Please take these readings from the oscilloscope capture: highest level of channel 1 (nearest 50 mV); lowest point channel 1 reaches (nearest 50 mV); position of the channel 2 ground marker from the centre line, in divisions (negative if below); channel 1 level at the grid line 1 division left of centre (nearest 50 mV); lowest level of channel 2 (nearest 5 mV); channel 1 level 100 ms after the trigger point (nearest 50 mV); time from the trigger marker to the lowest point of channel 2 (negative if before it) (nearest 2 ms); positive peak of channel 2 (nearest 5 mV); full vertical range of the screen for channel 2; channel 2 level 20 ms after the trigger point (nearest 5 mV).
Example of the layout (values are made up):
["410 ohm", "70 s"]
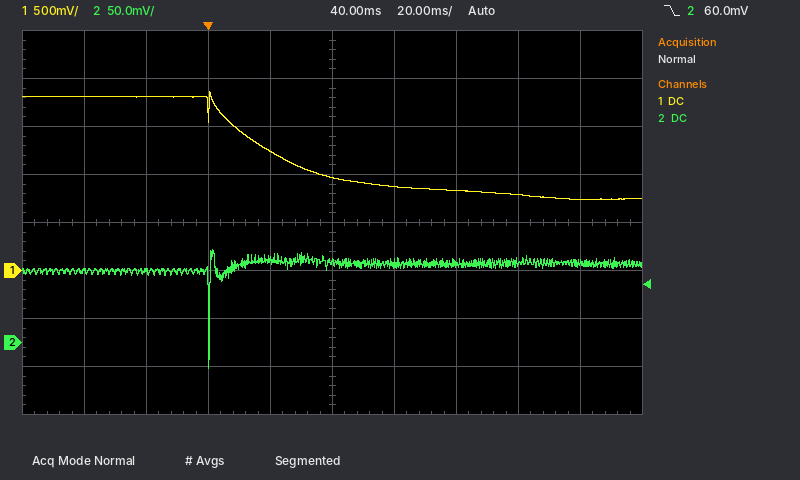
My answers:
["1.85 V", "750 mV", "-2.5 div", "1.25 V", "-25 mV", "800 mV", "0 ms", "95 mV", "400 mV", "85 mV"]
